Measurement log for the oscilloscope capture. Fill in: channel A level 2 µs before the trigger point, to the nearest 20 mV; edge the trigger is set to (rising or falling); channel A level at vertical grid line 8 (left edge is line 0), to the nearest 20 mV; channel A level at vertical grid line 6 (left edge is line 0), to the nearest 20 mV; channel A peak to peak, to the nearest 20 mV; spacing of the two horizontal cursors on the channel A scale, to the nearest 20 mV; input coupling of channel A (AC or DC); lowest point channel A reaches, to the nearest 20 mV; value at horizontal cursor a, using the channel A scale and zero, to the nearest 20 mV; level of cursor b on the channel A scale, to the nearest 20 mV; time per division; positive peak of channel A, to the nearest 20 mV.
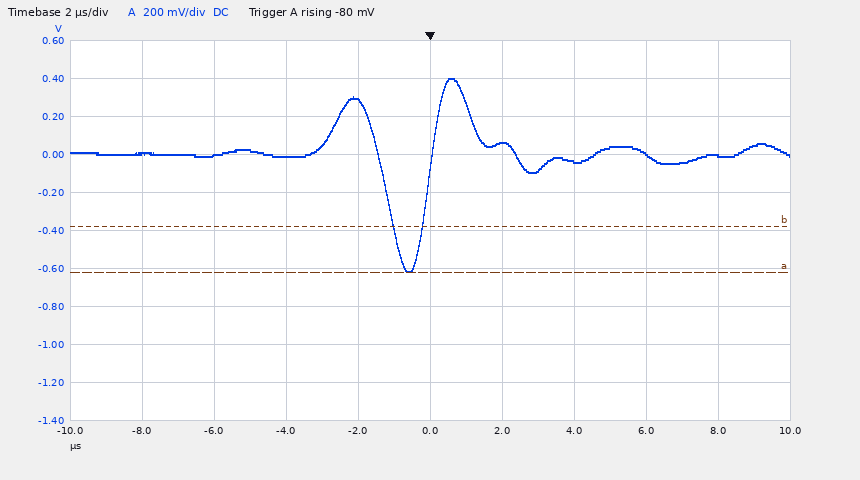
280 mV
rising
0 mV
60 mV
1.02 V
240 mV
DC
-620 mV
-620 mV
-380 mV
2 µs
400 mV
